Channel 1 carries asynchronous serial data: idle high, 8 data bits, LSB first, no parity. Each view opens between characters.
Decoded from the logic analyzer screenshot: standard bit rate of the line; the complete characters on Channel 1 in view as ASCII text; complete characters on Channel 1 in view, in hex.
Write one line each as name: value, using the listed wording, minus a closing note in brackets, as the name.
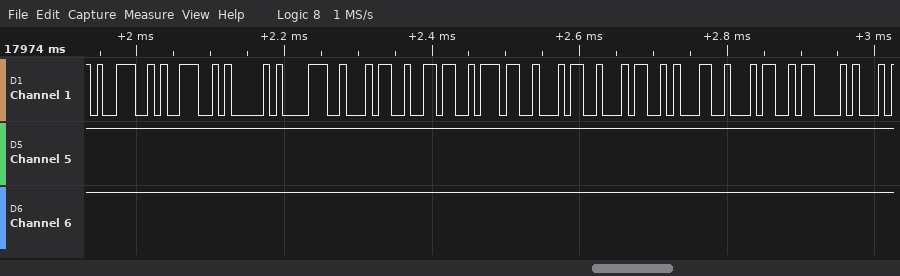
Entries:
standard bit rate of the line: 115200 baud
the complete characters on Channel 1 in view as ASCII text: "99A84674414C"
complete characters on Channel 1 in view, in hex: 39, 39, 41, 38, 34, 36, 37, 34, 34, 31, 34, 43
